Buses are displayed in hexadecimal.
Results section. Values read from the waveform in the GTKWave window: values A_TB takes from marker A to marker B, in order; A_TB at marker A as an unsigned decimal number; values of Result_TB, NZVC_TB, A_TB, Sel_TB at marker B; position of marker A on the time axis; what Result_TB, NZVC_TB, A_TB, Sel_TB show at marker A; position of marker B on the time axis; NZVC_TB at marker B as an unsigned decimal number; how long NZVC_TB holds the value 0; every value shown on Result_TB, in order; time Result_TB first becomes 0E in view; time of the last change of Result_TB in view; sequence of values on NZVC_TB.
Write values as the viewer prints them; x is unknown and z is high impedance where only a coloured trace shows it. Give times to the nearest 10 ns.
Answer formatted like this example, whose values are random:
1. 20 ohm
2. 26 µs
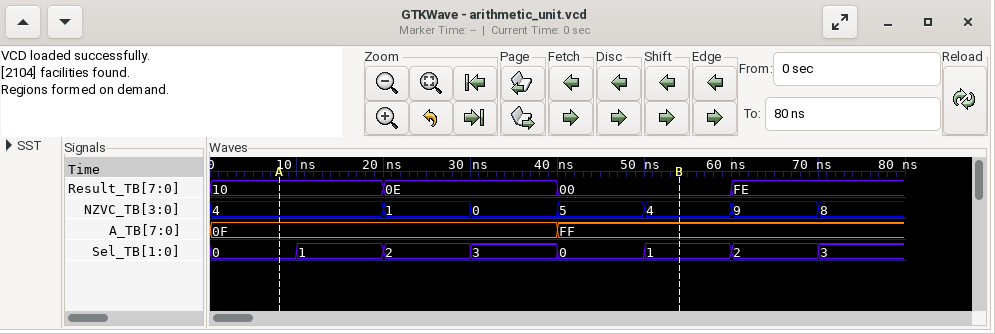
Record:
1. 0F, FF
2. 15
3. Result_TB=00, NZVC_TB=4, A_TB=FF, Sel_TB=1
4. 10 ns
5. Result_TB=10, NZVC_TB=4, A_TB=0F, Sel_TB=0
6. 50 ns
7. 4
8. 10 ns
9. 10, 0E, 00, FE
10. 20 ns
11. 60 ns
12. 4, 1, 0, 5, 4, 9, 8
